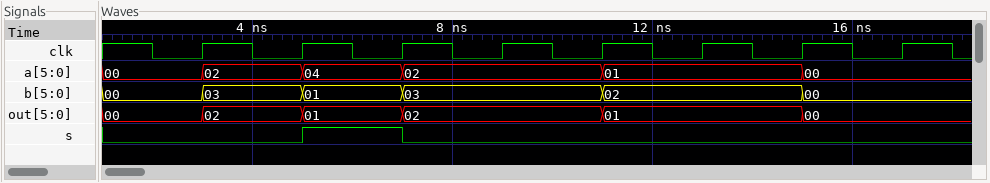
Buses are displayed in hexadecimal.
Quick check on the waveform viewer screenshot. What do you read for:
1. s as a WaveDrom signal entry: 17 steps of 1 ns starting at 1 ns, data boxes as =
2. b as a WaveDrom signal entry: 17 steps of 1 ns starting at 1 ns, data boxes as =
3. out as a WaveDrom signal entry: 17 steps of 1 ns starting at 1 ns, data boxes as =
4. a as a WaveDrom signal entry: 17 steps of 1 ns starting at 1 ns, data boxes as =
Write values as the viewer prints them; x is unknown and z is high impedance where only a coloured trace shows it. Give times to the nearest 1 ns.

{name: 's', wave: '0...1.0..........'}
{name: 'b', wave: '=.=.=.=...=...=..', data: '00 03 01 03 02 00'}
{name: 'out', wave: '=.=.=.=...=...=..', data: '00 02 01 02 01 00'}
{name: 'a', wave: '=.=.=.=...=...=..', data: '00 02 04 02 01 00'}
